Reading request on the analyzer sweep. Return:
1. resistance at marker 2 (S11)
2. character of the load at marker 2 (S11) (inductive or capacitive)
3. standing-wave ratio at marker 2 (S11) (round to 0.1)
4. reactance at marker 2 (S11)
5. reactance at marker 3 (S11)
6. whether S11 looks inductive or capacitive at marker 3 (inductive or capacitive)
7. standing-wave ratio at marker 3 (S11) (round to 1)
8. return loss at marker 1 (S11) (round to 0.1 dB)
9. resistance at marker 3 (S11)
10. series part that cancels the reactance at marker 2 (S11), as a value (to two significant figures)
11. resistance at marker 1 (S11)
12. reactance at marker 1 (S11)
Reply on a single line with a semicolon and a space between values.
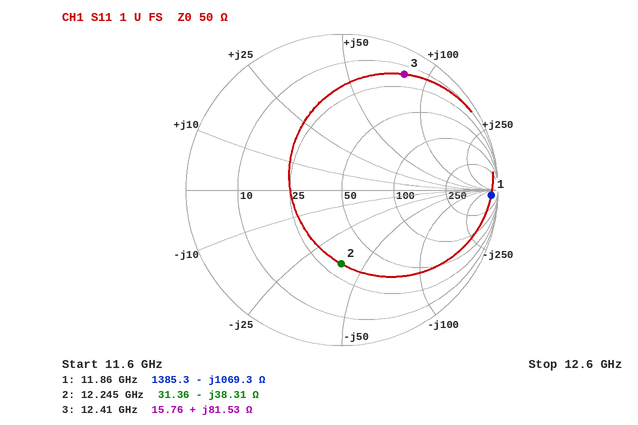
31.36 Ω; capacitive; 2.8; -38.31 Ω; +81.53 Ω; inductive; 12; 0.4 dB; 15.76 Ω; 500 pH; 1385.3 Ω; -1069.3 Ω
